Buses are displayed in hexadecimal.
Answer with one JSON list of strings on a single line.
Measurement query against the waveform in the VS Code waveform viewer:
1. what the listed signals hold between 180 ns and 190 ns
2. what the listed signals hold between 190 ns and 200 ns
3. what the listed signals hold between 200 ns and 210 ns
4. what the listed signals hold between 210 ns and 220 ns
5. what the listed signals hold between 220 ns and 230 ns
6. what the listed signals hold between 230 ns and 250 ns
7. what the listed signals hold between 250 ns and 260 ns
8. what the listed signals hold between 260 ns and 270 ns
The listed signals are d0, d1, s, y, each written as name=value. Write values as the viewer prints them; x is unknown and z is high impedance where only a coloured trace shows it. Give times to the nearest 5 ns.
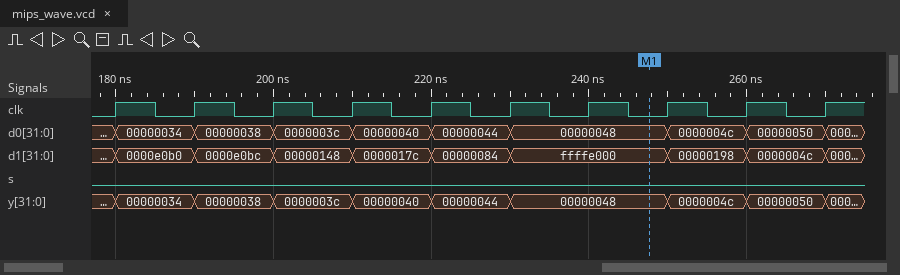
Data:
["d0=00000034, d1=0000e0b0, s=0, y=00000034", "d0=00000038, d1=0000e0bc, s=0, y=00000038", "d0=0000003c, d1=00000148, s=0, y=0000003c", "d0=00000040, d1=0000017c, s=0, y=00000040", "d0=00000044, d1=00000084, s=0, y=00000044", "d0=00000048, d1=ffffe000, s=0, y=00000048", "d0=0000004c, d1=00000198, s=0, y=0000004c", "d0=00000050, d1=0000004c, s=0, y=00000050"]
